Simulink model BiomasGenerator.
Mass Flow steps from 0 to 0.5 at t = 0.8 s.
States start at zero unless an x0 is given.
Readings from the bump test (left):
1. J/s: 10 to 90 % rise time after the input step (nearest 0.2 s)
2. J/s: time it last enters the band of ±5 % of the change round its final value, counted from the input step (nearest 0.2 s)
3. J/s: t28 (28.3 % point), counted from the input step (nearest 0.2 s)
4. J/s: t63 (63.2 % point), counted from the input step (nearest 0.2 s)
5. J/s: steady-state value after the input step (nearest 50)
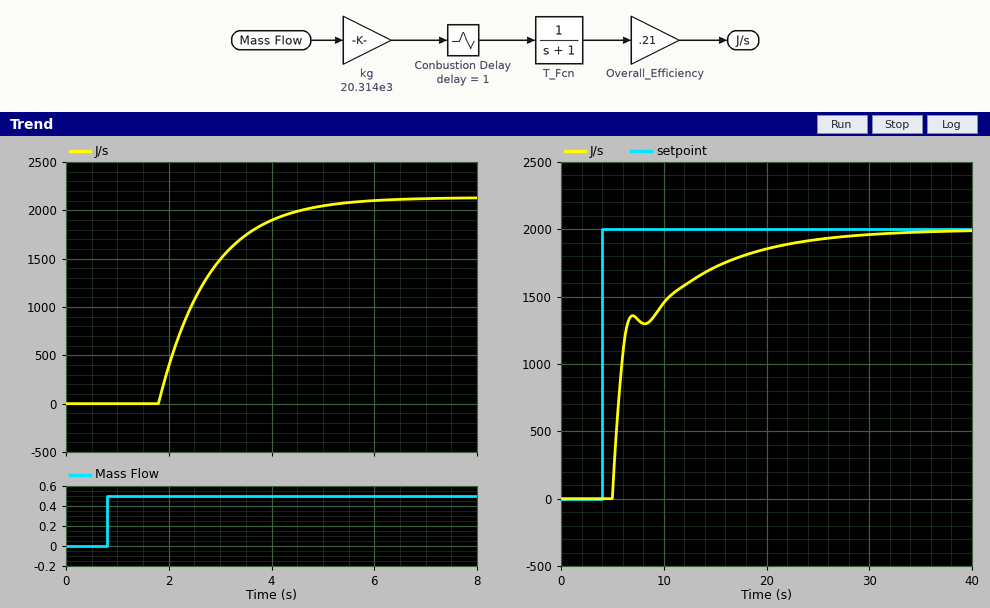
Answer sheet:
2.2 s
4.0 s
1.4 s
2.0 s
2150
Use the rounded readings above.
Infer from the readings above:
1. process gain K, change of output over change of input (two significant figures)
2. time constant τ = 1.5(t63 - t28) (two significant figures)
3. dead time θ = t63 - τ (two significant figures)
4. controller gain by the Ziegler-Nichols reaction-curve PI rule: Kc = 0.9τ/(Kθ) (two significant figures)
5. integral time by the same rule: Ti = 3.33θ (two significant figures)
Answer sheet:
4300
0.90 s
1.1 s
0.00017
3.7 s
